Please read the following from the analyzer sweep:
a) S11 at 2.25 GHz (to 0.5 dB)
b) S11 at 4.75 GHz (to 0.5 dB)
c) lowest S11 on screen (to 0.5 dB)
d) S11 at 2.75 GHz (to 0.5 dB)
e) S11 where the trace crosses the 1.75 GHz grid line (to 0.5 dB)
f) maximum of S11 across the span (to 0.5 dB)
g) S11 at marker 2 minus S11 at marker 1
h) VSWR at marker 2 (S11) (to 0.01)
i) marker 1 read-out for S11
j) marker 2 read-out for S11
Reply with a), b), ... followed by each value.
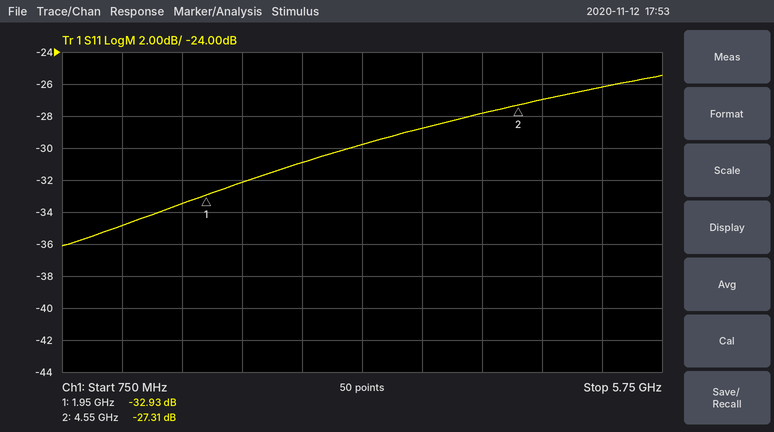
a) -32.0 dB
b) -27.0 dB
c) -36.0 dB
d) -31.0 dB
e) -33.5 dB
f) -25.5 dB
g) 5.62 dB
h) 1.09
i) -32.93 dB
j) -27.31 dB
